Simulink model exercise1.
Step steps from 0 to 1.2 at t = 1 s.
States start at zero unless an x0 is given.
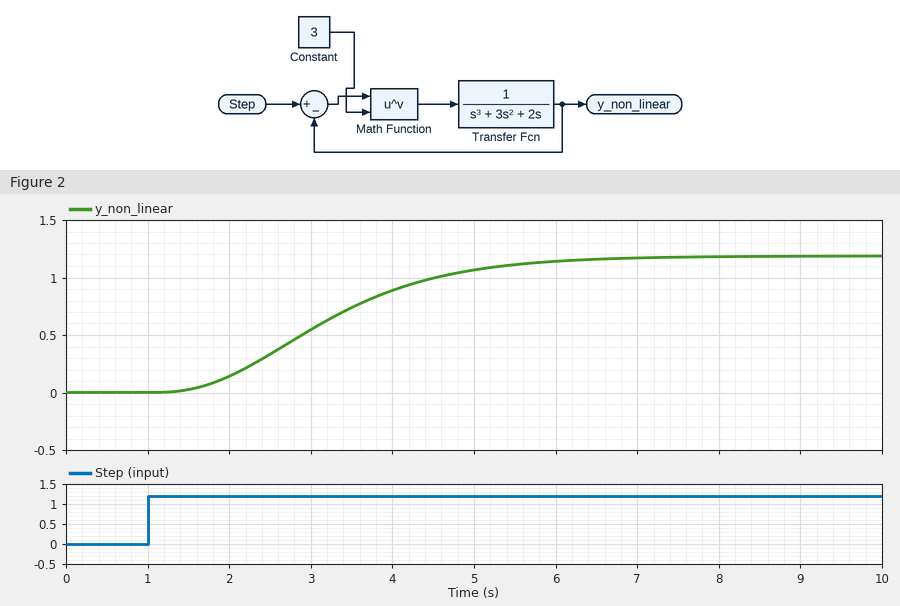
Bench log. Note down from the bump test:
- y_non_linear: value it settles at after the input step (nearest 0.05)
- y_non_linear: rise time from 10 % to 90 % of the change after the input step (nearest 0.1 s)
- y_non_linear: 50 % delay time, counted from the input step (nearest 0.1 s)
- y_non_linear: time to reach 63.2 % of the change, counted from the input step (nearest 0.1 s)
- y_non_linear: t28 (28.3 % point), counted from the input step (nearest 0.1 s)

1.20
3.1 s
2.1 s
2.5 s
1.5 s
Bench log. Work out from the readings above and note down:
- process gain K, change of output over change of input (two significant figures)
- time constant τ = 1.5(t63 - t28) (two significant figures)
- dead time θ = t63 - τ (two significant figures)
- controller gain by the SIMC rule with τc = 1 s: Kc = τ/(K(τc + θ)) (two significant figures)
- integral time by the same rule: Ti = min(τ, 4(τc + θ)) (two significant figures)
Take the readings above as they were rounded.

1.0
1.5 s
1.0 s
0.75
1.5 s
